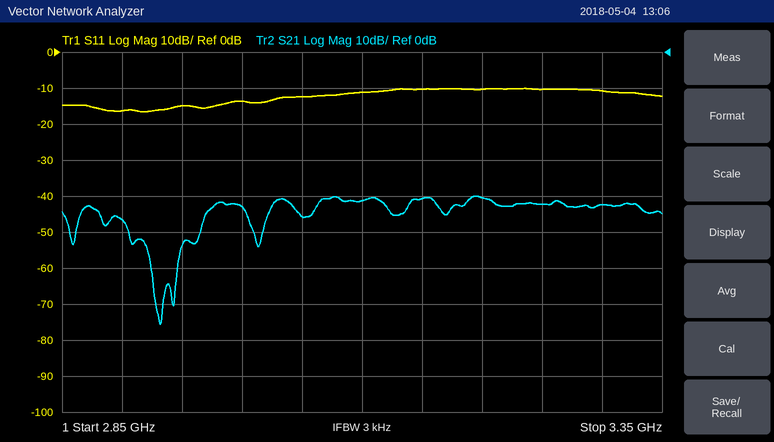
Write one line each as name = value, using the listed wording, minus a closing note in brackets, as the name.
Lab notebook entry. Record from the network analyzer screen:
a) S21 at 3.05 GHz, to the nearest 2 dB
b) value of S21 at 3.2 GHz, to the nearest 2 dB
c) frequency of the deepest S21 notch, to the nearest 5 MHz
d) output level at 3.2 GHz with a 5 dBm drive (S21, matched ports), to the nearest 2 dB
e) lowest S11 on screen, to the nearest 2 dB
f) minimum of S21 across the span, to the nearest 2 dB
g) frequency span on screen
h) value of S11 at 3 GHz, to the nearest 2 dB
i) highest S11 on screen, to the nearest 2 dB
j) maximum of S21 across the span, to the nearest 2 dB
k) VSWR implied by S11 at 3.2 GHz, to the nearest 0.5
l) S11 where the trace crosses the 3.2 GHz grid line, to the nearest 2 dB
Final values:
S21 at 3.05 GHz, to the nearest 2 dB = -46 dB
value of S21 at 3.2 GHz, to the nearest 2 dB = -40 dB
frequency of the deepest S21 notch, to the nearest 5 MHz = 2.930 GHz
output level at 3.2 GHz with a 5 dBm drive (S21, matched ports), to the nearest 2 dB = -36 dBm
lowest S11 on screen, to the nearest 2 dB = -16 dB
minimum of S21 across the span, to the nearest 2 dB = -76 dB
frequency span on screen = 500 MHz
value of S11 at 3 GHz, to the nearest 2 dB = -14 dB
highest S11 on screen, to the nearest 2 dB = -10 dB
maximum of S21 across the span, to the nearest 2 dB = -40 dB
VSWR implied by S11 at 3.2 GHz, to the nearest 0.5 = 2.0
S11 where the trace crosses the 3.2 GHz grid line, to the nearest 2 dB = -10 dB
